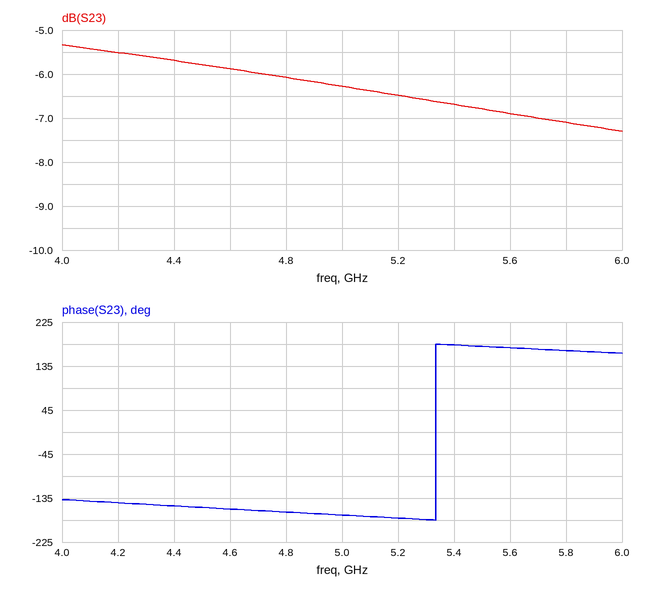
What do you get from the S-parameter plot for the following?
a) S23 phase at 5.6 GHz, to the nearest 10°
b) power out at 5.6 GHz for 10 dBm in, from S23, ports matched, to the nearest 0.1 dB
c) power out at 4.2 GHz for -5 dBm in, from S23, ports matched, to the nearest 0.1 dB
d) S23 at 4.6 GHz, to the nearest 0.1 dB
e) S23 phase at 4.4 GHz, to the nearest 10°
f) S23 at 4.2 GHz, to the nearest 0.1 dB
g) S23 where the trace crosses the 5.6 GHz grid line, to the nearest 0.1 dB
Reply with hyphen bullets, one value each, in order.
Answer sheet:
- 170°
- 3.1 dBm
- -10.5 dBm
- -5.9 dB
- -150°
- -5.5 dB
- -6.9 dB
